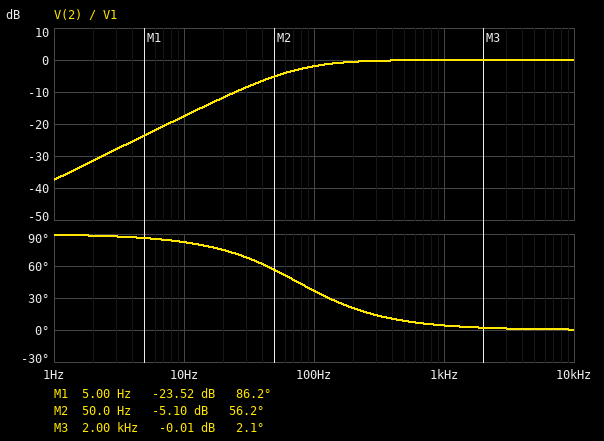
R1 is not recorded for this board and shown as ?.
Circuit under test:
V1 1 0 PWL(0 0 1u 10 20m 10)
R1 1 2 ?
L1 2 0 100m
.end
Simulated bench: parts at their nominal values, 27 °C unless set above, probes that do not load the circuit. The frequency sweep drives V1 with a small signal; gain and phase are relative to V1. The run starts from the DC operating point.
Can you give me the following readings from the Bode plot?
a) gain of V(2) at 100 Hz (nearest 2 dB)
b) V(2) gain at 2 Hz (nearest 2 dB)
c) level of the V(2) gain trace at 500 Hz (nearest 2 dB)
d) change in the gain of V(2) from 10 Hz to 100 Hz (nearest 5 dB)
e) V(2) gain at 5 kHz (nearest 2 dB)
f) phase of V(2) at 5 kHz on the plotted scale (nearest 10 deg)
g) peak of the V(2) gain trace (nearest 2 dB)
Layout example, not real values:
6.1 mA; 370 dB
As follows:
-2 dB; -32 dB; 0 dB; 15 dB; 0 dB; 0 deg; 0 dB
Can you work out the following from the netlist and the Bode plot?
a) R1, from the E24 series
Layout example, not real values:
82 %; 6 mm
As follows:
47 Ω
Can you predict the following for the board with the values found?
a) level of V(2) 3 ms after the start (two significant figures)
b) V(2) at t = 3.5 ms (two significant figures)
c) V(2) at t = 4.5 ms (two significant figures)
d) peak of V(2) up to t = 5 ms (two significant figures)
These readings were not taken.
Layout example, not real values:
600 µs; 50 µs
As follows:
2.4 V; 1.9 V; 1.2 V; 10 V
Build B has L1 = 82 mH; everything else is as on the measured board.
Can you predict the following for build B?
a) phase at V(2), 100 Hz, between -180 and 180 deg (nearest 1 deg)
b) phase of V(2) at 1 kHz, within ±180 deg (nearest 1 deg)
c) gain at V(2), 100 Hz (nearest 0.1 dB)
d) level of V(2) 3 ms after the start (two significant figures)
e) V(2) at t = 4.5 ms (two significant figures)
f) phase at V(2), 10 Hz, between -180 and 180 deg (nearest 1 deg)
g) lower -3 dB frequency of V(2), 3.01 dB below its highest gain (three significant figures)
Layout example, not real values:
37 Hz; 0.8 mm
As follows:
42 deg; 5 deg; -2.6 dB; 1.8 V; 760 mV; 84 deg; 91.2 Hz
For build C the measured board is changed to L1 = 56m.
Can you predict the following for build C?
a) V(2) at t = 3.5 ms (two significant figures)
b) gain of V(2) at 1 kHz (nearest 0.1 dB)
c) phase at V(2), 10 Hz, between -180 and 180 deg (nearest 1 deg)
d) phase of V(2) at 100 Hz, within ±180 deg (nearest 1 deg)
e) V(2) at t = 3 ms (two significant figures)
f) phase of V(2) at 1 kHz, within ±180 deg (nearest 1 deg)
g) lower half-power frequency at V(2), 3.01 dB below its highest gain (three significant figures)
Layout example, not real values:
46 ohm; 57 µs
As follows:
530 mV; -0.1 dB; 86 deg; 53 deg; 810 mV; 8 deg; 134 Hz
